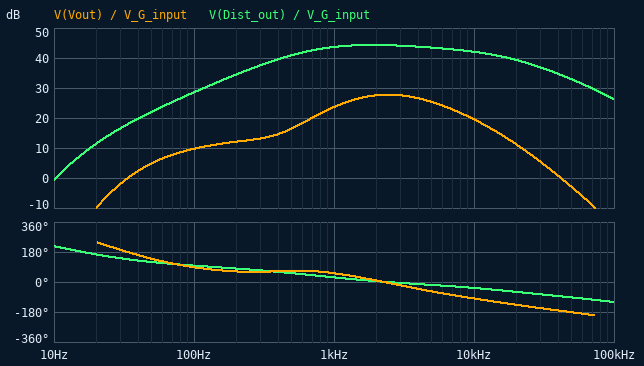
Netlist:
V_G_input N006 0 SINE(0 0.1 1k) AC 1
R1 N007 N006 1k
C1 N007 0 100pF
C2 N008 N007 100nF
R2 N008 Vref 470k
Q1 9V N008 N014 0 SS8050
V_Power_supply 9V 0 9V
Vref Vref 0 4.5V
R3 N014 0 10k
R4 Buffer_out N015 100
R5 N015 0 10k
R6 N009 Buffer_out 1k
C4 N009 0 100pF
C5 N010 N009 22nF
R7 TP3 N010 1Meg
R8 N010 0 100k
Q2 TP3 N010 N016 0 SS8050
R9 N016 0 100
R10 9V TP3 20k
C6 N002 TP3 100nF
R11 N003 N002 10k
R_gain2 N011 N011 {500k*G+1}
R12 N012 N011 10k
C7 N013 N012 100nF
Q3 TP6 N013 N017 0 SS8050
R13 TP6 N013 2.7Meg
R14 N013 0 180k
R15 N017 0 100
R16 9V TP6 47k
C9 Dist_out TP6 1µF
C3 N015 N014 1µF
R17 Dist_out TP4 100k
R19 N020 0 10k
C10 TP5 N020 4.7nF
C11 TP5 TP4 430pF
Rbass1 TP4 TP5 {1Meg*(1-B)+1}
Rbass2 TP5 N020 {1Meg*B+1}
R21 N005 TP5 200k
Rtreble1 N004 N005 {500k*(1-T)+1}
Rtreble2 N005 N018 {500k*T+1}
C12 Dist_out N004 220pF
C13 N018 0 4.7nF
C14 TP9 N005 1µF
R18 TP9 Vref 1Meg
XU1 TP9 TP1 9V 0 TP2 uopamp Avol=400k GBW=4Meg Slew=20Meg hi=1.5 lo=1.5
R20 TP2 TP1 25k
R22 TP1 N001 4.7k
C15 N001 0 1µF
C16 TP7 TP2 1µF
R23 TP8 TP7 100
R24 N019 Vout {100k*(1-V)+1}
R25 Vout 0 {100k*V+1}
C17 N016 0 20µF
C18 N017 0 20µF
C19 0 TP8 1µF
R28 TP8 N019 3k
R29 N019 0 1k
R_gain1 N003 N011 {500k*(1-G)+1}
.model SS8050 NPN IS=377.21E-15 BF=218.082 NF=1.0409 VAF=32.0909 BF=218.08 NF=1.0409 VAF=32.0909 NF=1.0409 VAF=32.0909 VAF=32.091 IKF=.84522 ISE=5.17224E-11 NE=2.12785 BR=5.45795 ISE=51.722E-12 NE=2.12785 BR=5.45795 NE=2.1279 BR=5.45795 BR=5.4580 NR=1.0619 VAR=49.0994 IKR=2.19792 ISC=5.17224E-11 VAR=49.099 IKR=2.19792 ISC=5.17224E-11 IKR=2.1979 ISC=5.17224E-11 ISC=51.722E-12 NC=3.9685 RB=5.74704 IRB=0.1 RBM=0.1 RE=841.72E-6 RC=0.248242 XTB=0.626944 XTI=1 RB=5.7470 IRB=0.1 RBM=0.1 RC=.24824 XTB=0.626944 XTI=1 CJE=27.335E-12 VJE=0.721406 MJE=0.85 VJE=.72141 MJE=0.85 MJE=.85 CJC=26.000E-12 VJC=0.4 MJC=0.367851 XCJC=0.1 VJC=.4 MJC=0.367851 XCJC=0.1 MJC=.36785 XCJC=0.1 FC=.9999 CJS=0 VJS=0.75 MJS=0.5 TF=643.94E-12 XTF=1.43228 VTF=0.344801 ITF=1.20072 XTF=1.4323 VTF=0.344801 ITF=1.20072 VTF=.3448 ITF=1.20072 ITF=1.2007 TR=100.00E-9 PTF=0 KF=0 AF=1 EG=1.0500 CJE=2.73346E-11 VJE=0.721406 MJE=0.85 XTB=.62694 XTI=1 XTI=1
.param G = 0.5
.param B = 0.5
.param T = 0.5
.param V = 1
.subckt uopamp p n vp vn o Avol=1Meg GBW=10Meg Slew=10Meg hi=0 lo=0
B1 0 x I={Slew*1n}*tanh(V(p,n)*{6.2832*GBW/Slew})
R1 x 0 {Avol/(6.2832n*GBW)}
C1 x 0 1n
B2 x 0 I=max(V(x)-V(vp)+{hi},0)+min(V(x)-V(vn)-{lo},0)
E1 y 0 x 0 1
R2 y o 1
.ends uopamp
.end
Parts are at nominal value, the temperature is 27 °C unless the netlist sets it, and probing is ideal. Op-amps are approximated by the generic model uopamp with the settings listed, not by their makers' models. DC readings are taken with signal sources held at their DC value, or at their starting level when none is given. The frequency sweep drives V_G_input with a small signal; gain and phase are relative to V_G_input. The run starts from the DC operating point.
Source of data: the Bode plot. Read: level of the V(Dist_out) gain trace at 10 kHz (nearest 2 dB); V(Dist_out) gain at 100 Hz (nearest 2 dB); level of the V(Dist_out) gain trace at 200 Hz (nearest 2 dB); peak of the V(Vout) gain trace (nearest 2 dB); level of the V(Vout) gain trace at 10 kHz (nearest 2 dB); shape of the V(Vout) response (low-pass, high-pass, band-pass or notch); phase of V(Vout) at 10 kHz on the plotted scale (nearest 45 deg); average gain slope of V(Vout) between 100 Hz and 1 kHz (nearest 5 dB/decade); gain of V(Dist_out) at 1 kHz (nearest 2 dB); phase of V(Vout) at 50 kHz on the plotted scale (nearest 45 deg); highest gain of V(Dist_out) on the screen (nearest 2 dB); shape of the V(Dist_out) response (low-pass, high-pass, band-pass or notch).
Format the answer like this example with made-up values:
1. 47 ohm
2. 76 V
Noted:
1. 42 dB
2. 28 dB
3. 34 dB
4. 28 dB
5. 20 dB
6. band-pass
7. -90 deg
8. 15 dB/decade
9. 44 dB
10. -180 deg
11. 44 dB
12. band-pass
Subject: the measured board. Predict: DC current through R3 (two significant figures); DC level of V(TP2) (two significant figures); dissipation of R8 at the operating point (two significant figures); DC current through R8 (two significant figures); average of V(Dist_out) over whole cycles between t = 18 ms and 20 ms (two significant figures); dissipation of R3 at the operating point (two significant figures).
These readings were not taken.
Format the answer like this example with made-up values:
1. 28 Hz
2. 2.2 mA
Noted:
1. 290 µA
2. 4.5 V
3. 2.8 µW
4. 5.3 µA
5. -4.4 V
6. 850 µW
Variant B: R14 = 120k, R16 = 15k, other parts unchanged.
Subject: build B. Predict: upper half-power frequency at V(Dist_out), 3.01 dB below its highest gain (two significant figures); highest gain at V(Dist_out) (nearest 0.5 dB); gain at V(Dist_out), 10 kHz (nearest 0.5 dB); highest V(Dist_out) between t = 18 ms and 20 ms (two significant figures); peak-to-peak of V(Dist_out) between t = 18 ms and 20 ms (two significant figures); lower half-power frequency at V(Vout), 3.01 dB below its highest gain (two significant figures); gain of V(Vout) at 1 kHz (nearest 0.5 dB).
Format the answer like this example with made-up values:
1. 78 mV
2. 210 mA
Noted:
1. 30 kHz
2. 12.0 dB
3. 11.5 dB
4. 43 mV
5. 5.1 V
6. 1.2 kHz
7. -9.0 dB
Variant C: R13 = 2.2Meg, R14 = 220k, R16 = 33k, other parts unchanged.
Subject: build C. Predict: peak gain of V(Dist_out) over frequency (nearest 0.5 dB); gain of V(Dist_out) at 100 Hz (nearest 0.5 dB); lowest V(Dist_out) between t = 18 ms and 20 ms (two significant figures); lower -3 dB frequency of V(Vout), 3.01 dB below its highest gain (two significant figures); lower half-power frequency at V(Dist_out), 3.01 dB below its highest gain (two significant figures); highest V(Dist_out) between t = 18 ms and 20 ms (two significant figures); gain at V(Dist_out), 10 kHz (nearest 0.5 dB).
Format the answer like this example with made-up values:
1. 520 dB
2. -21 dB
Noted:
1. 46.5 dB
2. 30.5 dB
3. -6.8 V
4. 1.2 kHz
5. 570 Hz
6. 1.7 V
7. 44.5 dB
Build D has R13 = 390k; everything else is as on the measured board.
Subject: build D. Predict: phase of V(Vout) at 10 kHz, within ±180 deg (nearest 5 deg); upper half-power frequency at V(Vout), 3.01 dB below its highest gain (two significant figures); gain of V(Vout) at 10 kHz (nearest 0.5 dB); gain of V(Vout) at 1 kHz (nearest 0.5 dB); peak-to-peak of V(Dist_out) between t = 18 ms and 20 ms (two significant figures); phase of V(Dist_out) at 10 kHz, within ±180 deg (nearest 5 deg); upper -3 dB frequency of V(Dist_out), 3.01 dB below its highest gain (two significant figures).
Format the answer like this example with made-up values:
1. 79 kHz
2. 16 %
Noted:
1. -80 deg
2. 6.4 kHz
3. 14.0 dB
4. 15.5 dB
5. 7.4 V
6. -20 deg
7. 31 kHz
